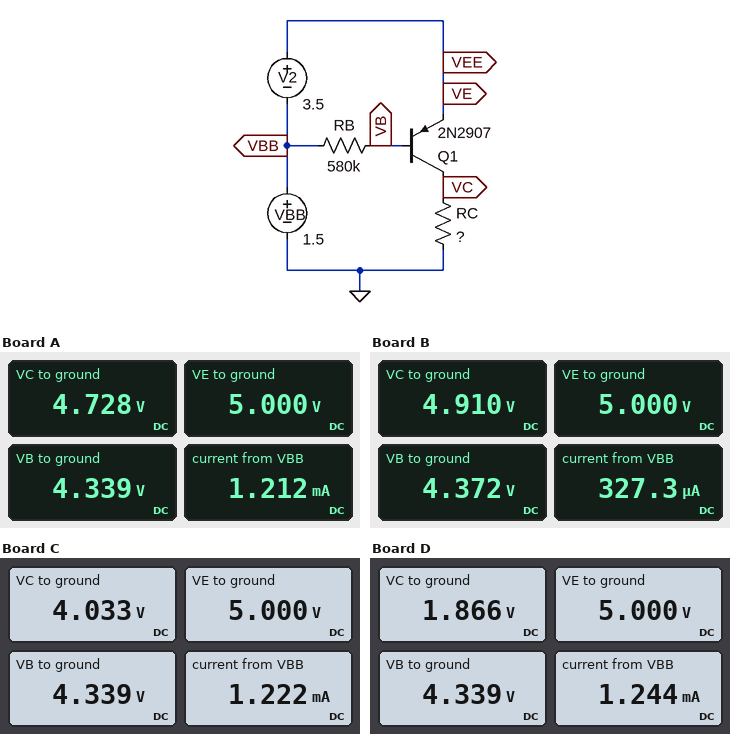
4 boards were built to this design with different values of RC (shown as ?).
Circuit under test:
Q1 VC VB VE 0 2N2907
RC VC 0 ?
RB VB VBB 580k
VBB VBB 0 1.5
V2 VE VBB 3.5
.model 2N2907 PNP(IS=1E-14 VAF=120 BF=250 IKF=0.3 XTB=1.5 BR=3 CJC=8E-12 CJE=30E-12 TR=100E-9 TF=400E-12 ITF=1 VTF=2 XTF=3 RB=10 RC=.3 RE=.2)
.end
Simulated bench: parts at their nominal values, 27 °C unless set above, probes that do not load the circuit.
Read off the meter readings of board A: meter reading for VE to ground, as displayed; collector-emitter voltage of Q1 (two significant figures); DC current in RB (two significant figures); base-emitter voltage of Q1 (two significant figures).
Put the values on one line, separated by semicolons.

5.000 V; -270 mV; 4.9 µA; -660 mV
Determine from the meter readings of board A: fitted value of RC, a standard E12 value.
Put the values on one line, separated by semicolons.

3.9 kΩ
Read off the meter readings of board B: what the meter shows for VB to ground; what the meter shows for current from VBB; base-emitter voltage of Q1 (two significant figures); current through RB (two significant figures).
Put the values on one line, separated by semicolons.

4.372 V; 327.3 µA; -630 mV; 5.0 µA
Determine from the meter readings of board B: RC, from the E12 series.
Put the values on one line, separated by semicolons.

15 kΩ
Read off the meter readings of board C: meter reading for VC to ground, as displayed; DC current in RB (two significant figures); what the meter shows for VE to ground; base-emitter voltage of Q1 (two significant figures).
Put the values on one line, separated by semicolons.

4.033 V; 4.9 µA; 5.000 V; -660 mV
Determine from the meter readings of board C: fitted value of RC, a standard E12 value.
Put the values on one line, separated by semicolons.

3.3 kΩ
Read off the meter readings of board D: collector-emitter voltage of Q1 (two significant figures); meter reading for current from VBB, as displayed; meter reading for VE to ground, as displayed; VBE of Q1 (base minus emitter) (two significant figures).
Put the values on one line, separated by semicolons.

-3.1 V; 1.244 mA; 5.000 V; -660 mV
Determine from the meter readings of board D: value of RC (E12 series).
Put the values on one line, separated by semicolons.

1.5 kΩ
